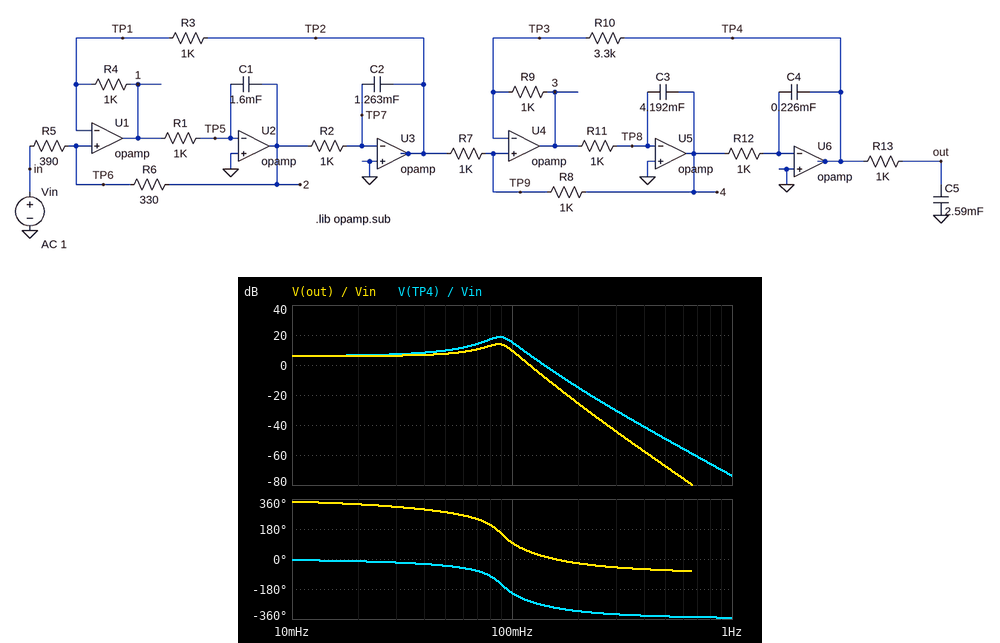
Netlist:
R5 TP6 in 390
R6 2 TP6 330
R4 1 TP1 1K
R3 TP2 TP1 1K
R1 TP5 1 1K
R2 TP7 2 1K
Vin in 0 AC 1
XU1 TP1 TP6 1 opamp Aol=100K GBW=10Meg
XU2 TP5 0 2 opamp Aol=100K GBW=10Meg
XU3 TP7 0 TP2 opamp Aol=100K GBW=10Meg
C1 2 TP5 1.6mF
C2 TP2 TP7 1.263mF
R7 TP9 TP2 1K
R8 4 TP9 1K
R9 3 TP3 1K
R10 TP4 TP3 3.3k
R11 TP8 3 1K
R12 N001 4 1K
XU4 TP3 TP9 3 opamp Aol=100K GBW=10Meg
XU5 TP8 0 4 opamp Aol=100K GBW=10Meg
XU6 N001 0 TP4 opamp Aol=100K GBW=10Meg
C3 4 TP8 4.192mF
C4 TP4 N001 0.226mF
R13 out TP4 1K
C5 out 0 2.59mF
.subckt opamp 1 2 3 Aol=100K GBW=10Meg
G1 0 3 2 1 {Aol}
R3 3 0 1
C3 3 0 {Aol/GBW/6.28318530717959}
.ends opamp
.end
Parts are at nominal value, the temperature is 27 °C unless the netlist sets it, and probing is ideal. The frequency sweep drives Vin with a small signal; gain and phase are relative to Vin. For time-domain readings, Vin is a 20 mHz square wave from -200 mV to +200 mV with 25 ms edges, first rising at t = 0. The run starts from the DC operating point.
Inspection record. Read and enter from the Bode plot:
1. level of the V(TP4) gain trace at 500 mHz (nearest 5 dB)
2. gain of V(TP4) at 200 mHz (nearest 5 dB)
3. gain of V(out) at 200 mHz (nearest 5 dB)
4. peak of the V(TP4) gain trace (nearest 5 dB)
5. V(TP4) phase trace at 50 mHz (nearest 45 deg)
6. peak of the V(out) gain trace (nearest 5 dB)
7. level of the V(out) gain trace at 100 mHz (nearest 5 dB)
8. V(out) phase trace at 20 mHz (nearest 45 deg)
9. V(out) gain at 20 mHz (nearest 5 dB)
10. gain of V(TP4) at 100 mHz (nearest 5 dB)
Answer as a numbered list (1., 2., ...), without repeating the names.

1. -50 dB
2. -15 dB
3. -25 dB
4. 20 dB
5. -45 deg
6. 15 dB
7. 10 dB
8. 315 deg
9. 5 dB
10. 15 dB
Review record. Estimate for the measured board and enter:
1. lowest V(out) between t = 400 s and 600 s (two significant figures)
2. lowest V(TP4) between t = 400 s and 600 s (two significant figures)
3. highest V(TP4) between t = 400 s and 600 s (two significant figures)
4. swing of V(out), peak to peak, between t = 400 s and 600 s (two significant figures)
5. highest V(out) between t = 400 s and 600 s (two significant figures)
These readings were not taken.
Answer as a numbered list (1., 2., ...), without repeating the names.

1. -690 mV
2. -970 mV
3. 970 mV
4. 1.4 V
5. 690 mV
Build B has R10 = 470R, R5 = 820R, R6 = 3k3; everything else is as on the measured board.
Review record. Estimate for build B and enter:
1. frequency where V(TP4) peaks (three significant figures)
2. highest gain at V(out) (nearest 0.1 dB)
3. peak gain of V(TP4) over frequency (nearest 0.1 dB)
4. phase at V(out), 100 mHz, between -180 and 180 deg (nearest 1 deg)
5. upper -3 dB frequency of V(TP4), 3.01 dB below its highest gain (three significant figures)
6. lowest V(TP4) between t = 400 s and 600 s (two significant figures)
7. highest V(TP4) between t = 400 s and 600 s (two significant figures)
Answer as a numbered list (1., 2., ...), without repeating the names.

1. 110 mHz
2. 6.4 dB
3. 12.5 dB
4. -123 deg
5. 131 mHz
6. -640 mV
7. 640 mV
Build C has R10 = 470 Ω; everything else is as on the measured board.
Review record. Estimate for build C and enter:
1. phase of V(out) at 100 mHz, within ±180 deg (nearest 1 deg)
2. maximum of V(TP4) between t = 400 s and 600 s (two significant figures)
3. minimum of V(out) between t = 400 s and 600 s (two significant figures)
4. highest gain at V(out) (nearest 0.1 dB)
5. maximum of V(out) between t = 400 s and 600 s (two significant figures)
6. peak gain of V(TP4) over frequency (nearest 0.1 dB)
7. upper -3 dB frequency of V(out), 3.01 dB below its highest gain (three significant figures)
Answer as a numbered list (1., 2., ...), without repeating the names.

1. -142 deg
2. 220 mV
3. -140 mV
4. -3.4 dB
5. 140 mV
6. -0.7 dB
7. 101 mHz
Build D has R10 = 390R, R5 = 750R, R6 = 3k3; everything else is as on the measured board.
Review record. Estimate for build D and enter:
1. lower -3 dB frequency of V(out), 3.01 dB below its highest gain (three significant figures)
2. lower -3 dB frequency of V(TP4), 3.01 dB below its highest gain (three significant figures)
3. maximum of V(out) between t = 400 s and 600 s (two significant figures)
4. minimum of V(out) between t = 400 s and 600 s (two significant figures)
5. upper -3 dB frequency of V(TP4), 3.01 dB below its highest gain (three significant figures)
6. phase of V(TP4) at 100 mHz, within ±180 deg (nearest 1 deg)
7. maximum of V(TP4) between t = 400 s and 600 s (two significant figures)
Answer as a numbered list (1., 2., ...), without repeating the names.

1. 83.0 mHz
2. 91.0 mHz
3. 330 mV
4. -330 mV
5. 129 mHz
6. -62 deg
7. 590 mV
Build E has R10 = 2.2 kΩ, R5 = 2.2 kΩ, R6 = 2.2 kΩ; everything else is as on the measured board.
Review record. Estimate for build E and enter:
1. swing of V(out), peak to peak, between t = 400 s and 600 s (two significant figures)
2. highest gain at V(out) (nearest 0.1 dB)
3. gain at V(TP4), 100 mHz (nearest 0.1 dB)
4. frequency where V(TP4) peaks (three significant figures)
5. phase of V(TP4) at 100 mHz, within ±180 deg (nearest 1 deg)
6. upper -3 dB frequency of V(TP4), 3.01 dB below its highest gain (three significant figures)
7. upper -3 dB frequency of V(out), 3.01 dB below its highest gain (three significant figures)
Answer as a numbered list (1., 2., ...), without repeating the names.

1. 1.1 V
2. 11.5 dB
3. 16.6 dB
4. 107 mHz
5. -128 deg
6. 119 mHz
7. 117 mHz
